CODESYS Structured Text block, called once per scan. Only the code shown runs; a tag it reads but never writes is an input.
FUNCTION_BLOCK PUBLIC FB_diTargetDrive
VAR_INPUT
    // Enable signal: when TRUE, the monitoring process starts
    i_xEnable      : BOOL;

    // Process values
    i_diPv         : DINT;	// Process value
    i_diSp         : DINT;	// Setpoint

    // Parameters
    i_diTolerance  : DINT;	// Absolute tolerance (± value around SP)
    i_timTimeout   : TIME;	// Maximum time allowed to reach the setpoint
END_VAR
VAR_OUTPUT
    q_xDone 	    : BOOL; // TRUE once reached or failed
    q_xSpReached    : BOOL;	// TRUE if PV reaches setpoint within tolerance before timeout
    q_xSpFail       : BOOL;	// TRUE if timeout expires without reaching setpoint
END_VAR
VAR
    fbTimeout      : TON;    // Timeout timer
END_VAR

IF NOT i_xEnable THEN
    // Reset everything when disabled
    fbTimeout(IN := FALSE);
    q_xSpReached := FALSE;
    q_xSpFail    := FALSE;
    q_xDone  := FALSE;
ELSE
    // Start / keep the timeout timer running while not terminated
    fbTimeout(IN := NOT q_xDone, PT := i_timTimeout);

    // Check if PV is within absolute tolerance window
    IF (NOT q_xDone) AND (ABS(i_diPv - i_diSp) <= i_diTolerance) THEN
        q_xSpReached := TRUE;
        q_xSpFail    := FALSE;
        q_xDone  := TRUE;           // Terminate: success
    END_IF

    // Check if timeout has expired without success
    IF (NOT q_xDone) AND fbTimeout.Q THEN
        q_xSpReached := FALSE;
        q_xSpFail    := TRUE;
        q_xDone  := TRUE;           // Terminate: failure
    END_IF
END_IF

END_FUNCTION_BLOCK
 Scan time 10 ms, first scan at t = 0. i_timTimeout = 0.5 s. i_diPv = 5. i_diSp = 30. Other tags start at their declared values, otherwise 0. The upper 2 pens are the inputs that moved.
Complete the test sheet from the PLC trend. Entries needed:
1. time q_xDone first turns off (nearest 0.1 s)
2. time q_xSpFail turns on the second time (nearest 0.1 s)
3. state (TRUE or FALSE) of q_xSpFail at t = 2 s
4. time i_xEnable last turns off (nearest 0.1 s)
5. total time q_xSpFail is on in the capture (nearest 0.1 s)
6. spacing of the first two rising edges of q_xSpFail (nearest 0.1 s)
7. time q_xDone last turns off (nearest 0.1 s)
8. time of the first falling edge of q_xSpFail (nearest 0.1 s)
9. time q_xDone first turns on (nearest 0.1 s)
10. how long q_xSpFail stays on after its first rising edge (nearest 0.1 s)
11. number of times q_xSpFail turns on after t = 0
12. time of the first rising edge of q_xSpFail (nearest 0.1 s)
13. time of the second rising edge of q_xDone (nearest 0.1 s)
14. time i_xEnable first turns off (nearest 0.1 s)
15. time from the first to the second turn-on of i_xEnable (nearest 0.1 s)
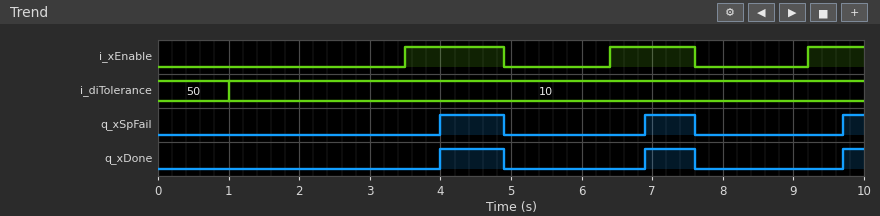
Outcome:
4.9 s
6.9 s
FALSE
7.6 s
1.9 s
2.9 s
7.6 s
4.9 s
4.0 s
0.9 s
3
4.0 s
6.9 s
4.9 s
2.9 s
